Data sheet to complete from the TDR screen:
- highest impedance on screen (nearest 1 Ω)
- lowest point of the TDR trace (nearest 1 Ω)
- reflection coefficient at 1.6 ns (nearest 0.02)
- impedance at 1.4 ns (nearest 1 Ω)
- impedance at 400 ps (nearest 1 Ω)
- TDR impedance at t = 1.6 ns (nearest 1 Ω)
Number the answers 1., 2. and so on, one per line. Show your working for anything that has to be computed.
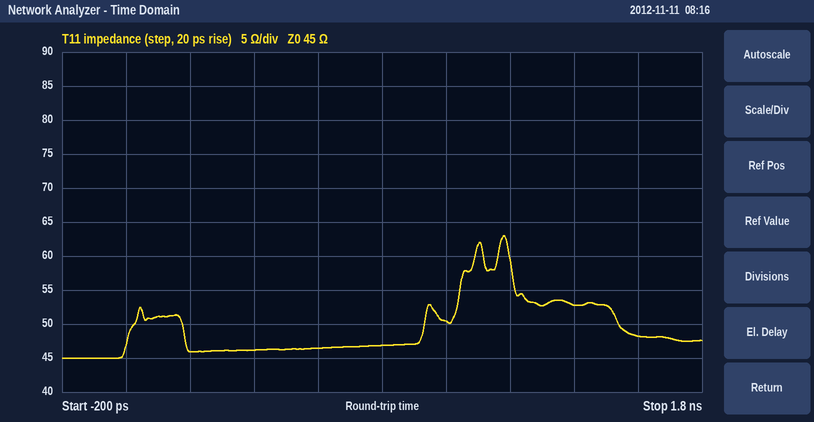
1. 63 Ω
2. 45 Ω
3. (48 − 45)/(48 + 45) ≈ +0.0323, so +0.04 to the nearest 0.02
4. 53 Ω
5. 46 Ω
6. 48 Ω
